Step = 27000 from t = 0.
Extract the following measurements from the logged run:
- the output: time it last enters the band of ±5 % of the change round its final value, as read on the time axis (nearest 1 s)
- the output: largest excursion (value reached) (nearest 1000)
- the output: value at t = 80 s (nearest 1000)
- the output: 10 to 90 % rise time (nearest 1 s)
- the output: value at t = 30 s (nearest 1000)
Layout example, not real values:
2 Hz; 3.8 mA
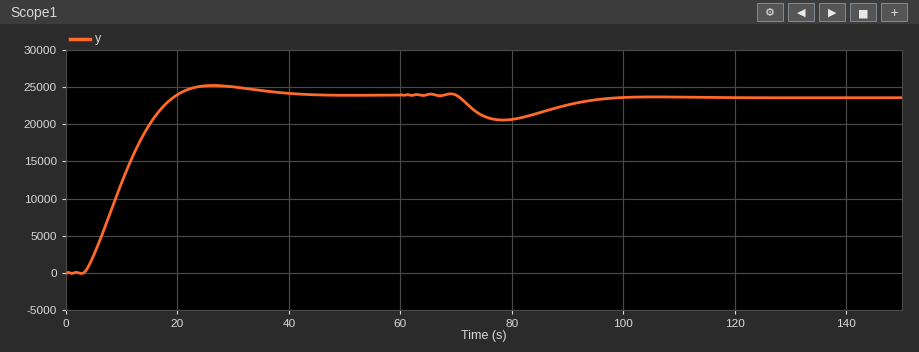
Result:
89 s; 25000; 21000; 11 s; 25000
